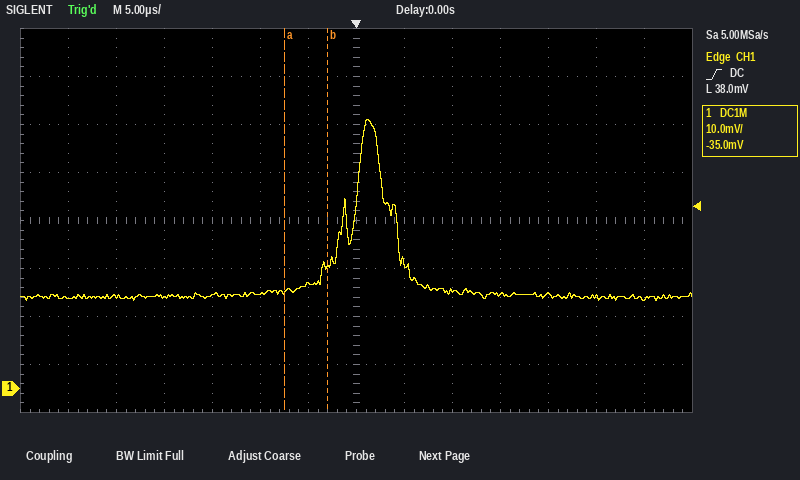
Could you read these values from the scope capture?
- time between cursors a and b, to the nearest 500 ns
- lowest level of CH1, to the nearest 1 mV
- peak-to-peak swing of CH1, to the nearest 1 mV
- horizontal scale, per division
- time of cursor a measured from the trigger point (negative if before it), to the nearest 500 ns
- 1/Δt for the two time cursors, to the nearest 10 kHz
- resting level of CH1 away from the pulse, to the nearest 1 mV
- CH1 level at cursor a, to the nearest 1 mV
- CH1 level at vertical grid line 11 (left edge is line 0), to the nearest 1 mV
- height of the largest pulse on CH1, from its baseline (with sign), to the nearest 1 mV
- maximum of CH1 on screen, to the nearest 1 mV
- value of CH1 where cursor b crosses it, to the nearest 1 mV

4.5 µs
18 mV
38 mV
5 µs
-7.5 µs
220 kHz
19 mV
20 mV
20 mV
+37 mV
56 mV
26 mV
